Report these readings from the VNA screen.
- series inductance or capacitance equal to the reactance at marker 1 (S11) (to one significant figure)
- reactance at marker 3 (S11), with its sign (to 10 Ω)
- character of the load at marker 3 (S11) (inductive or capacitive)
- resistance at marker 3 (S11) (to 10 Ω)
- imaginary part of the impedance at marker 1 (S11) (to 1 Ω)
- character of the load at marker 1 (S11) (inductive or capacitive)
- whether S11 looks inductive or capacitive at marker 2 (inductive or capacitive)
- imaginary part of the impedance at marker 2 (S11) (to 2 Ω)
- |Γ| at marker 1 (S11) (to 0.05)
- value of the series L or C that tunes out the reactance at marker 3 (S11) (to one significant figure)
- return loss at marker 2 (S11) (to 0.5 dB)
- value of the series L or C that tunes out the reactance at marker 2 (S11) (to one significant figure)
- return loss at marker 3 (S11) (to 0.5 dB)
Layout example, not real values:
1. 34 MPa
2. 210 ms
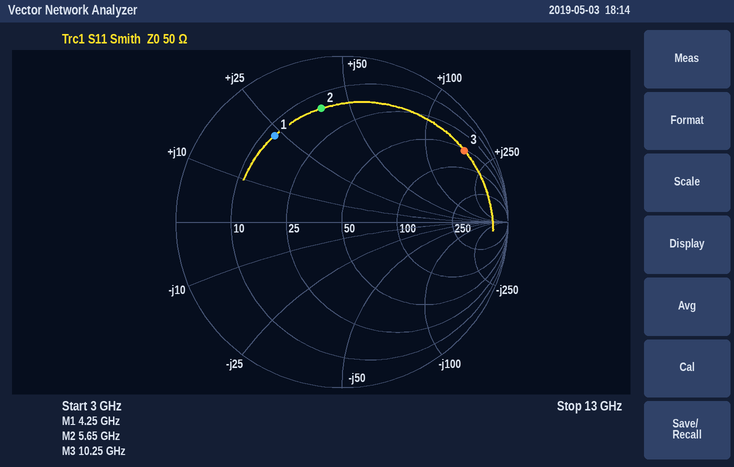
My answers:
1. 900 pH
2. +170 Ω
3. inductive
4. 50 Ω
5. +23 Ω
6. inductive
7. inductive
8. +40 Ω
9. 0.65
10. 90 fF
11. 3.0 dB
12. 700 fF
13. 1.5 dB
